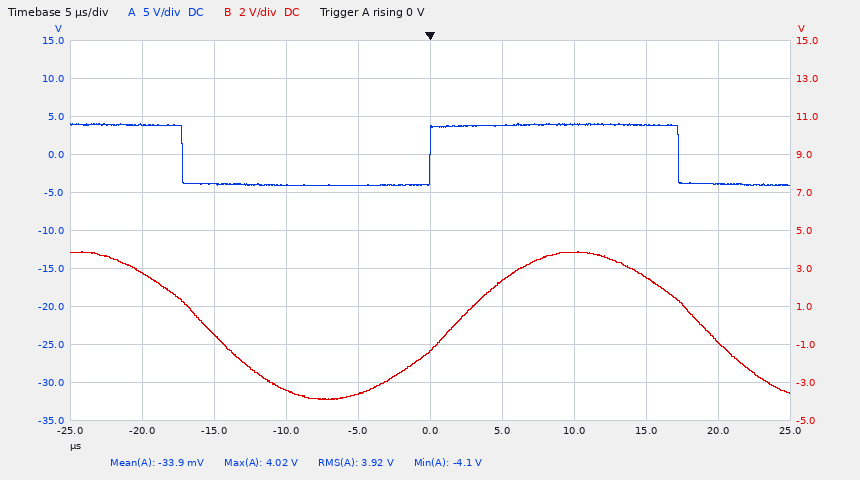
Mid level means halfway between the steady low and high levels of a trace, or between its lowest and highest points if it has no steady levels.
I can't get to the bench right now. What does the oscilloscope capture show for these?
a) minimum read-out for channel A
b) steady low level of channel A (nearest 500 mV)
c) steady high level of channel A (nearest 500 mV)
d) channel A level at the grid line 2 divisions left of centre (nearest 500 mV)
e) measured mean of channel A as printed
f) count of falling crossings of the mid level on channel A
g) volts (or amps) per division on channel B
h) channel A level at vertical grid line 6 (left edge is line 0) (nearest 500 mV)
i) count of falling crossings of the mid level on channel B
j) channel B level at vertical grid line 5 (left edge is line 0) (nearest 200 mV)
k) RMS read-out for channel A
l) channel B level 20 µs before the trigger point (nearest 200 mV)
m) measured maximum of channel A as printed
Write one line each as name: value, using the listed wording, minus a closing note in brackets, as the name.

minimum read-out for channel A: -4.1 V
steady low level of channel A: -4.0 V
steady high level of channel A: 4.0 V
channel A level at the grid line 2 divisions left of centre: -4.0 V
measured mean of channel A as printed: -33.9 mV
count of falling crossings of the mid level on channel A: 2
volts (or amps) per division on channel B: 2 V
channel A level at vertical grid line 6 (left edge is line 0): 4.0 V
count of falling crossings of the mid level on channel B: 2
channel B level at vertical grid line 5 (left edge is line 0): -1.4 V
RMS read-out for channel A: 3.92 V
channel B level 20 µs before the trigger point: 2.8 V
measured maximum of channel A as printed: 4.02 V
